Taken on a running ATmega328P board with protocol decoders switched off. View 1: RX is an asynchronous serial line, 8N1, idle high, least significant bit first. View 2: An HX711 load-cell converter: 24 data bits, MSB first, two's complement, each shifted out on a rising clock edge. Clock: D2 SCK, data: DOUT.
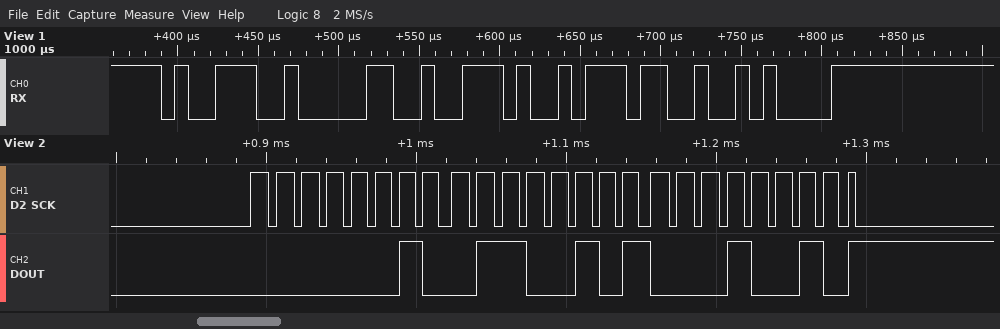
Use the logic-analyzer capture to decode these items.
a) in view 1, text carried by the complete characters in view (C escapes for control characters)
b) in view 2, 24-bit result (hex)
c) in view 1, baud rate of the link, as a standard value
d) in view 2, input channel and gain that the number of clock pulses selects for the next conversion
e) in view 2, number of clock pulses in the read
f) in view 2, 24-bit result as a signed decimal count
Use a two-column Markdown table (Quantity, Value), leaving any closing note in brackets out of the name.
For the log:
| Quantity | Value |
|---|---|
| in view 1, text carried by the complete characters in view | "90.7\n" |
| in view 2, 24-bit result | 0x026512 |
| in view 1, baud rate of the link, as a standard value | 115200 baud |
| in view 2, input channel and gain that the number of clock pulses selects for the next conversion | channel A, gain 128 |
| in view 2, number of clock pulses in the read | 25 |
| in view 2, 24-bit result as a signed decimal count | 156946 |
